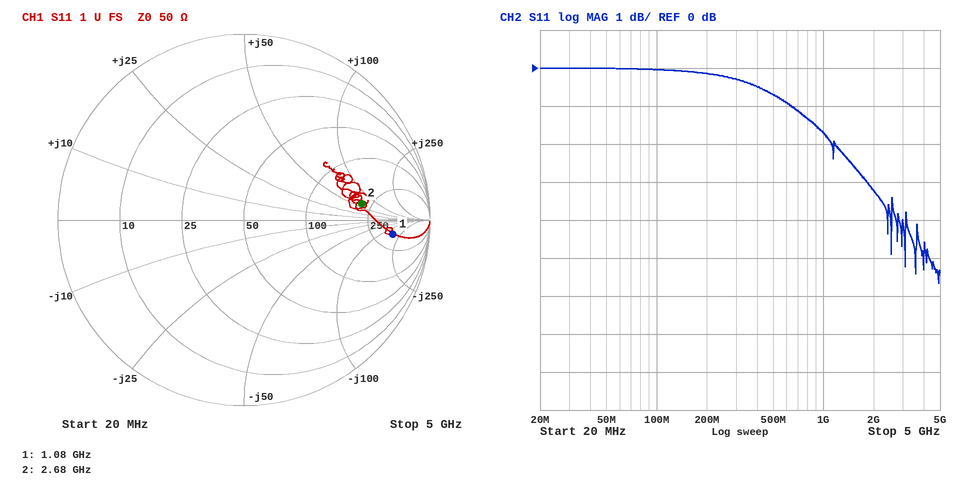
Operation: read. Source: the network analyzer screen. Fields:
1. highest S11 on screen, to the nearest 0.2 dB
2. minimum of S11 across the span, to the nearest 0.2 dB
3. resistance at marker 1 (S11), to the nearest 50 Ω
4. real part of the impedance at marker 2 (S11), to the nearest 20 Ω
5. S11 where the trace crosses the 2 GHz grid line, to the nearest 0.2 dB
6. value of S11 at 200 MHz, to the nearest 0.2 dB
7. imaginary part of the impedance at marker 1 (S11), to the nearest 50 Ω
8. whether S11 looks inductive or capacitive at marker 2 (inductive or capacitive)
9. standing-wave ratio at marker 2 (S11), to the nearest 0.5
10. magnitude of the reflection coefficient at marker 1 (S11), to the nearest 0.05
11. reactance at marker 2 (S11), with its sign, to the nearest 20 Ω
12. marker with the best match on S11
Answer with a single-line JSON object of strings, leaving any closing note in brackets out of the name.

{"highest S11 on screen, to the nearest 0.2 dB": "0.0 dB", "minimum of S11 across the span, to the nearest 0.2 dB": "-5.6 dB", "resistance at marker 1 (S11), to the nearest 50 Ω": "400 Ω", "real part of the impedance at marker 2 (S11), to the nearest 20 Ω": "200 Ω", "S11 where the trace crosses the 2 GHz grid line, to the nearest 0.2 dB": "-3.2 dB", "value of S11 at 200 MHz, to the nearest 0.2 dB": "-0.2 dB", "imaginary part of the impedance at marker 1 (S11), to the nearest 50 Ω": "-150 Ω", "whether S11 looks inductive or capacitive at marker 2": "inductive", "standing-wave ratio at marker 2 (S11), to the nearest 0.5": "4.5", "magnitude of the reflection coefficient at marker 1 (S11), to the nearest 0.05": "0.80", "reactance at marker 2 (S11), with its sign, to the nearest 20 Ω": "+60 Ω", "marker with the best match on S11": "marker 2"}
